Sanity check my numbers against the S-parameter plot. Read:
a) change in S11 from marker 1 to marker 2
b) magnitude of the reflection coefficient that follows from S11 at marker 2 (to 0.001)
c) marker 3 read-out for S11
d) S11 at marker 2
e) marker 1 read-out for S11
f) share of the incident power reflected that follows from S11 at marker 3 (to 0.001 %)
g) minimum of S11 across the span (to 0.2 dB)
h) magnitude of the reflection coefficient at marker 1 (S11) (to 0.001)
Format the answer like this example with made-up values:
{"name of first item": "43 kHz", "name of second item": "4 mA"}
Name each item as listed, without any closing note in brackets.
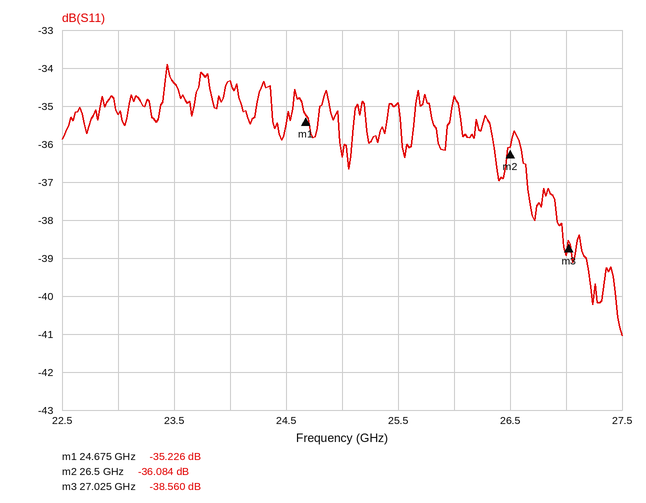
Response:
{"change in S11 from marker 1 to marker 2": "-0.858 dB", "magnitude of the reflection coefficient that follows from S11 at marker 2": "0.016", "marker 3 read-out for S11": "-38.560 dB", "S11 at marker 2": "-36.084 dB", "marker 1 read-out for S11": "-35.226 dB", "share of the incident power reflected that follows from S11 at marker 3": "0.014 %", "minimum of S11 across the span": "-41.0 dB", "magnitude of the reflection coefficient at marker 1 (S11)": "0.017"}
